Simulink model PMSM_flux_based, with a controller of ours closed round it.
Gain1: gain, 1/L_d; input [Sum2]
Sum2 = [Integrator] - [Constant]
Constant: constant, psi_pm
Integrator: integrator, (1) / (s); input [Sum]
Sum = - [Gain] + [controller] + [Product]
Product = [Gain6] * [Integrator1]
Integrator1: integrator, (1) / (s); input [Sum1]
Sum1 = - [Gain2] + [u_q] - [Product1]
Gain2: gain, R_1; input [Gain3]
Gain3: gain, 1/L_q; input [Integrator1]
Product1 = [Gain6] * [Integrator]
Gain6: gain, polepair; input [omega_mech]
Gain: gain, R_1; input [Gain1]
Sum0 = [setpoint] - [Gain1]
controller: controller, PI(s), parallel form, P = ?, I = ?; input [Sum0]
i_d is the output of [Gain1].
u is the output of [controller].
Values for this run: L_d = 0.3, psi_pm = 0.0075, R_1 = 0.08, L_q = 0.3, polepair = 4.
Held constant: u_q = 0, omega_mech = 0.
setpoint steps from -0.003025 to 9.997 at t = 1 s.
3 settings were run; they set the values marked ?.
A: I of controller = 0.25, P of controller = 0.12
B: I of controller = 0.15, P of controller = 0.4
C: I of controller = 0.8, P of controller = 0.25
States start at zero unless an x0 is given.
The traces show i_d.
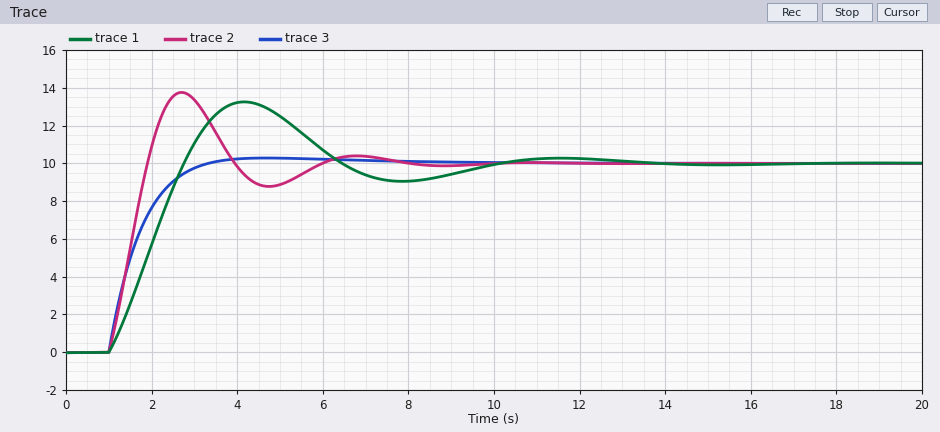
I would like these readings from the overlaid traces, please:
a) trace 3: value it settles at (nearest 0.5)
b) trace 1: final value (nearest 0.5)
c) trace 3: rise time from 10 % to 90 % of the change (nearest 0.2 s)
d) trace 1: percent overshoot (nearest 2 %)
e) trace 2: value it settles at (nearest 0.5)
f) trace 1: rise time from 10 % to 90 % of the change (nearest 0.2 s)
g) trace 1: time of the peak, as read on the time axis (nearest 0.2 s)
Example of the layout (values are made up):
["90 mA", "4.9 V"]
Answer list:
["10.0", "10.0", "1.4 s", "32 %", "10.0", "1.4 s", "4.2 s"]
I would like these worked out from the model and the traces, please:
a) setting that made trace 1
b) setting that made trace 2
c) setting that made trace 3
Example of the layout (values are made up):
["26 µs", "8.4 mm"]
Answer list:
["A", "C", "B"]
